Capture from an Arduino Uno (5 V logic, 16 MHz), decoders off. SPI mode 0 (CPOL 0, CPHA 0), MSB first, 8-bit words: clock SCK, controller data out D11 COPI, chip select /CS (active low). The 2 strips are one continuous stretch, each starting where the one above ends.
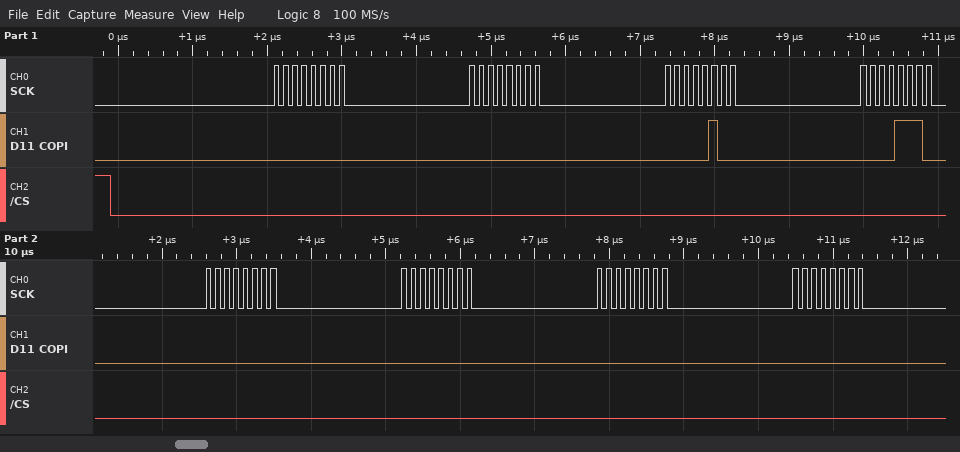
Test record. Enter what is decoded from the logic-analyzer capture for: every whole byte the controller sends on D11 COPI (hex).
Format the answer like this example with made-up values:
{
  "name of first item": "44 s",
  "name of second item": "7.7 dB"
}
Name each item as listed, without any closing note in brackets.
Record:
{
  "every whole byte the controller sends on D11 COPI": "00 00 04 0E 00 00 00 00"
}
